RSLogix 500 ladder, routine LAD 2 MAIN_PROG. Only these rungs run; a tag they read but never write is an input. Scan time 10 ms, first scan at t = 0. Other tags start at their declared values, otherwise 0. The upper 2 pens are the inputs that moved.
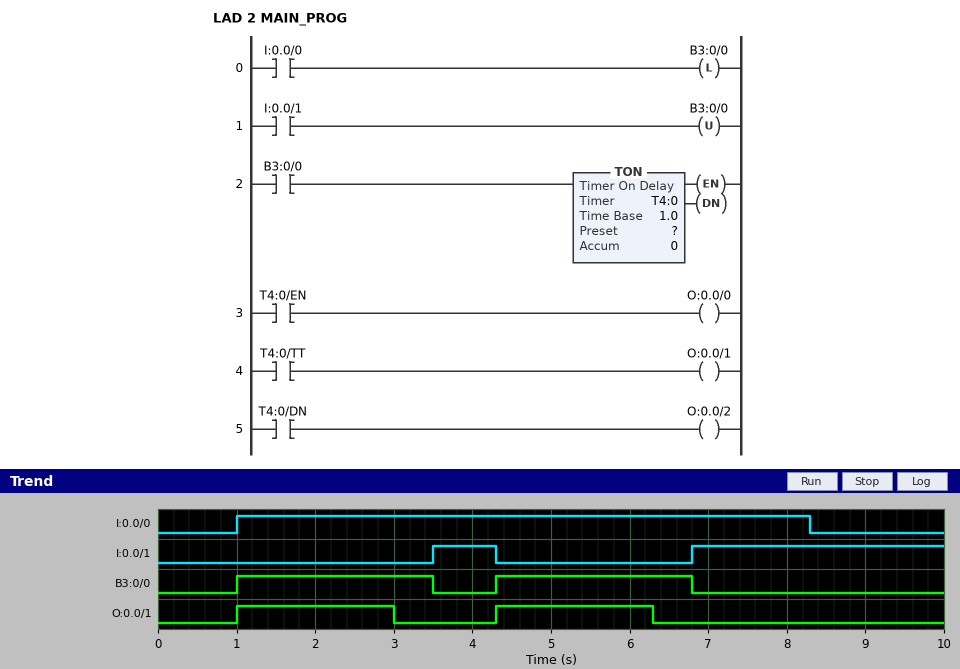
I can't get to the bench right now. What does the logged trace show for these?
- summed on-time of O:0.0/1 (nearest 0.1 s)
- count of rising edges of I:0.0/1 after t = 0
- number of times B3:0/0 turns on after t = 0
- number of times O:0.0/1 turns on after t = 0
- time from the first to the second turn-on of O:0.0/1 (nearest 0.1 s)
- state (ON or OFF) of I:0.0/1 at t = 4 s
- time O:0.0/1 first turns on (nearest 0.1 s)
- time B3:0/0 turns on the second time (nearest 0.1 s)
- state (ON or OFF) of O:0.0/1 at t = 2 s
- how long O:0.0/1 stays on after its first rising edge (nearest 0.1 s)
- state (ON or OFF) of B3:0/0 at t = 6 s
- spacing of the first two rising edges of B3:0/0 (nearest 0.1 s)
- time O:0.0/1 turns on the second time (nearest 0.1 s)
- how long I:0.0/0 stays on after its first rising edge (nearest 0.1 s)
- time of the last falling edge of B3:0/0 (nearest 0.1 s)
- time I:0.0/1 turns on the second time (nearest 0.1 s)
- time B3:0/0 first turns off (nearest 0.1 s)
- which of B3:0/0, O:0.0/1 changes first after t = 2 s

4.0 s
2
2
2
3.3 s
ON
1.0 s
4.3 s
ON
2.0 s
ON
3.3 s
4.3 s
7.3 s
6.8 s
6.8 s
3.5 s
O:0.0/1
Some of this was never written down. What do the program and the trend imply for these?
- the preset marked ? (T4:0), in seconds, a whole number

2 s
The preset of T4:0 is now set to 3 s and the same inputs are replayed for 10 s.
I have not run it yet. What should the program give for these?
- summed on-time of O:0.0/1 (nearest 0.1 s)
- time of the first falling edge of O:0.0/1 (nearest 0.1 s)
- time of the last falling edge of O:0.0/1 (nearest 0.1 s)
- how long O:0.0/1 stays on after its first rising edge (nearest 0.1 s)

5.0 s
3.5 s
6.8 s
2.5 s
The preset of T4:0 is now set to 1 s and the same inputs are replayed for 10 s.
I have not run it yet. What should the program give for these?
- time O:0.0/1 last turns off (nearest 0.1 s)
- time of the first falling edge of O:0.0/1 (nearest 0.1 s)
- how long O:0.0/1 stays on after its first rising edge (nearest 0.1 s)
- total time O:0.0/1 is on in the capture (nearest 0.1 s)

5.3 s
2.0 s
1.0 s
2.0 s
